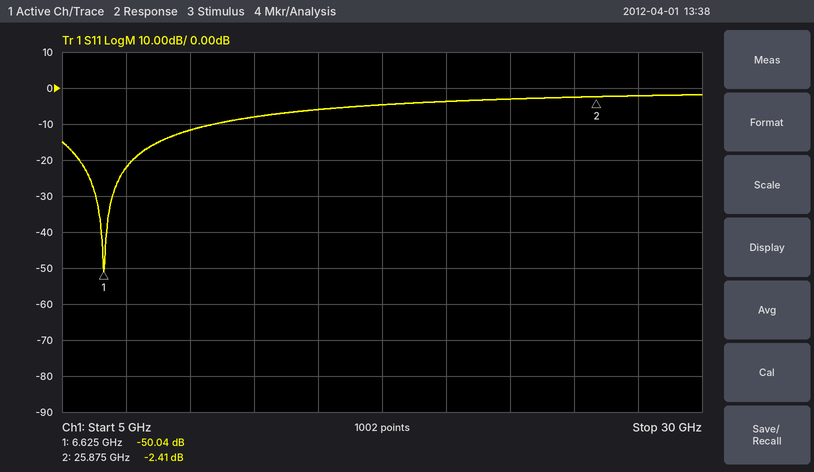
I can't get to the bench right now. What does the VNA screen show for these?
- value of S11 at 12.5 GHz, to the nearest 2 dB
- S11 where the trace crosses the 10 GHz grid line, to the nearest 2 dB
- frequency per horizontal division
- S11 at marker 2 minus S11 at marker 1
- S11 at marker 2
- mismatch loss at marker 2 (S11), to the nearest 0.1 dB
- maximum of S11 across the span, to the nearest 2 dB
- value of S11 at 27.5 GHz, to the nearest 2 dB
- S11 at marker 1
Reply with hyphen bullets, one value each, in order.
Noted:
- -8 dB
- -12 dB
- 2.5 GHz
- 47.63 dB
- -2.41 dB
- 3.7 dB
- -2 dB
- -2 dB
- -50.04 dB
